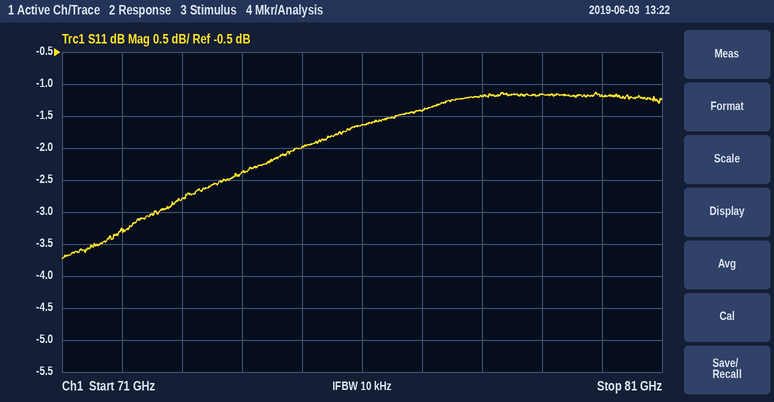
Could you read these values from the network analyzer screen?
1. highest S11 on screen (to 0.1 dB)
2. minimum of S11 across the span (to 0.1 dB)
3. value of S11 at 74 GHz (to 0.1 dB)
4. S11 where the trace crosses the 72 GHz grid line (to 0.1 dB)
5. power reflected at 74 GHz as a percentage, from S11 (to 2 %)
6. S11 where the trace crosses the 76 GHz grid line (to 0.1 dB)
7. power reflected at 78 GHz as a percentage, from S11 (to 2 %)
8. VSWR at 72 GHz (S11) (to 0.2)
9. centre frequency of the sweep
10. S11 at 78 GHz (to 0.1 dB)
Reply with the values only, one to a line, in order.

-1.1 dB
-3.7 dB
-2.4 dB
-3.3 dB
58 %
-1.6 dB
76 %
5.4
76 GHz
-1.2 dB
